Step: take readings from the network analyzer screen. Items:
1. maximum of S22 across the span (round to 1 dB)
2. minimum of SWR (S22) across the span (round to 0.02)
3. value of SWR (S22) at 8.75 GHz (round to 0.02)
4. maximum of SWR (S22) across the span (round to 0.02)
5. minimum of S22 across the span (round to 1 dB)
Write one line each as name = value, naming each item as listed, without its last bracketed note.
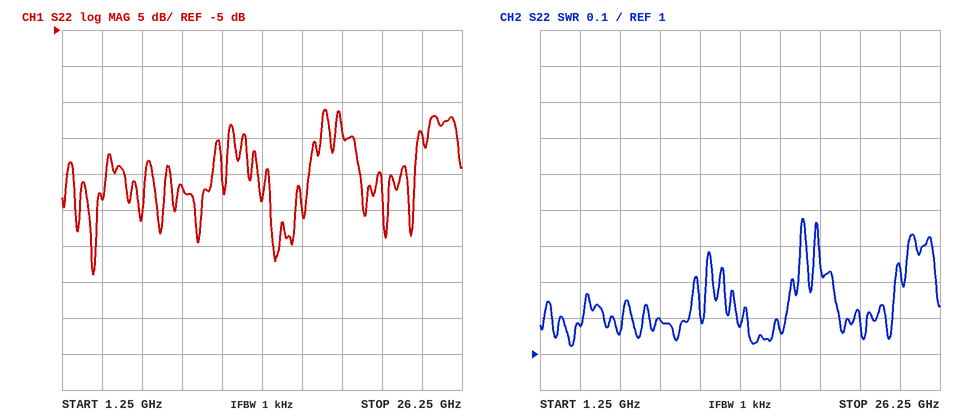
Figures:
maximum of S22 across the span = -16 dB
minimum of SWR (S22) across the span = 1.02
value of SWR (S22) at 8.75 GHz = 1.10
maximum of SWR (S22) across the span = 1.38
minimum of S22 across the span = -39 dB
